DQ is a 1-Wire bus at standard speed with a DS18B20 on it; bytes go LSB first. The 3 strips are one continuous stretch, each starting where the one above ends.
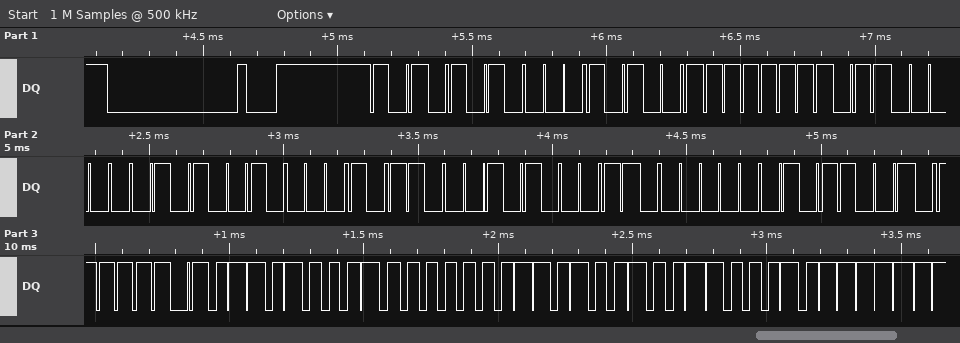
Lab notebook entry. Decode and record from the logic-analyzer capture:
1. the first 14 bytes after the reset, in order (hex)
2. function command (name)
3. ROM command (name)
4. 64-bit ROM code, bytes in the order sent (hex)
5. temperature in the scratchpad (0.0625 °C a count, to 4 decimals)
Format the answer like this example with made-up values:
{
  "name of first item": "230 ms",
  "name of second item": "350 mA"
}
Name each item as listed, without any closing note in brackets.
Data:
{
  "the first 14 bytes after the reset, in order": "55 28 FF 06 4A 68 14 03 9A BE 16 01 4B 46",
  "function command": "Read Scratchpad",
  "ROM command": "Match ROM",
  "64-bit ROM code, bytes in the order sent": "28 FF 06 4A 68 14 03 9A",
  "temperature in the scratchpad": "17.3750 °C"
}
